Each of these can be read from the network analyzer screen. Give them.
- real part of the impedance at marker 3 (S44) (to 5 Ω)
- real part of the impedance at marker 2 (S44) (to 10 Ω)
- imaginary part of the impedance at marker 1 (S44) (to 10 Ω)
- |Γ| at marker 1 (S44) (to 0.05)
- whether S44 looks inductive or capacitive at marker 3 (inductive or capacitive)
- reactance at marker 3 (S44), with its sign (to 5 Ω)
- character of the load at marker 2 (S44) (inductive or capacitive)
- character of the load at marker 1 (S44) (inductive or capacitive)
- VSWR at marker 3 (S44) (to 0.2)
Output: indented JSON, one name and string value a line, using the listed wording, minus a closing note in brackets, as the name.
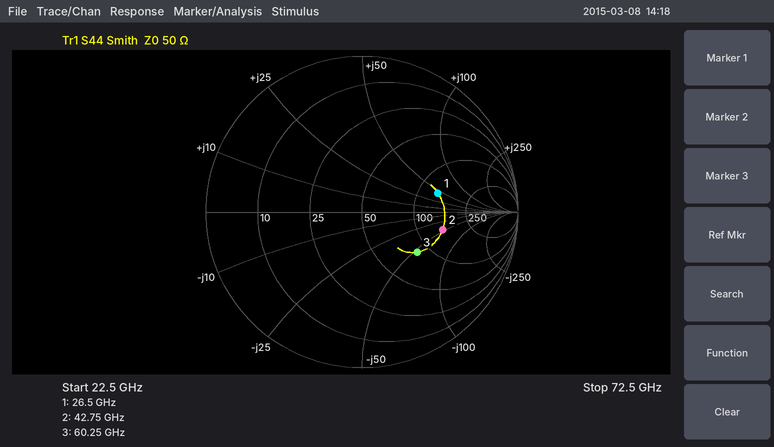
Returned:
{
  "real part of the impedance at marker 3 (S44)": "85 Ω",
  "real part of the impedance at marker 2 (S44)": "150 Ω",
  "imaginary part of the impedance at marker 1 (S44)": "+40 Ω",
  "|Γ| at marker 1 (S44)": "0.50",
  "whether S44 looks inductive or capacitive at marker 3": "capacitive",
  "reactance at marker 3 (S44), with its sign": "-55 Ω",
  "character of the load at marker 2 (S44)": "capacitive",
  "character of the load at marker 1 (S44)": "inductive",
  "VSWR at marker 3 (S44)": "2.6"
}
